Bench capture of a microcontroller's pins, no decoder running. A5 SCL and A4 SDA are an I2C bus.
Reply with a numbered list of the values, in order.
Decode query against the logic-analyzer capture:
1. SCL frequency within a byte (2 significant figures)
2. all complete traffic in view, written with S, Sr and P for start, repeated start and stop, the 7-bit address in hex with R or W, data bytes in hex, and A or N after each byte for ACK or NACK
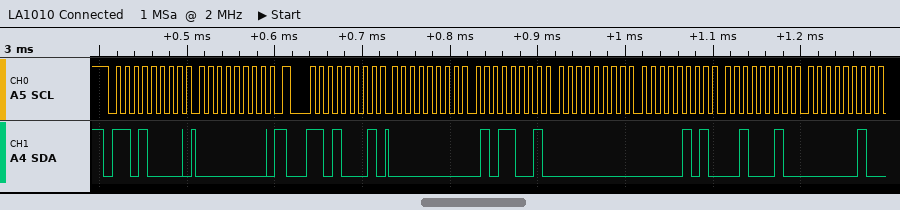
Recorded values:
1. 100 kHz
2. S 68W A 00 A Sr 68R A 00 A 59 A 00 A 05 A 22 A 02 A
